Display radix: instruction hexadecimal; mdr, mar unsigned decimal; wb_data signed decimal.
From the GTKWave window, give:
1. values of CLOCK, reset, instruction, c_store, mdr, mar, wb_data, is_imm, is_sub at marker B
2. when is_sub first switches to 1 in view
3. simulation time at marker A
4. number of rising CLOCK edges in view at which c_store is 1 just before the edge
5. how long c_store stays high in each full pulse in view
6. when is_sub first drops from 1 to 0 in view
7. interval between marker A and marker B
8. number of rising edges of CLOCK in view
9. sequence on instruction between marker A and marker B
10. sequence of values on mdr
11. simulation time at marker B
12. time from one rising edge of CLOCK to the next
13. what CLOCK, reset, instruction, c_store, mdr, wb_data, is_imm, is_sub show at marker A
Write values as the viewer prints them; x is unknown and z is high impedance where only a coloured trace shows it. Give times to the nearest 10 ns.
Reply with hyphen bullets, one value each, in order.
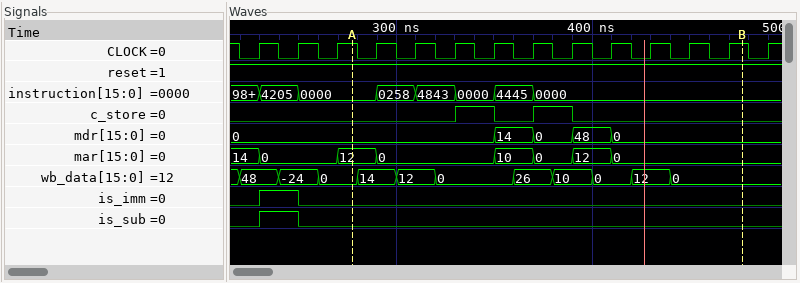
- CLOCK=1, reset=1, instruction=0000, c_store=0, mdr=0, mar=0, wb_data=0, is_imm=0, is_sub=0
- 230 ns
- 280 ns
- 2
- 20 ns, 20 ns
- 250 ns
- 200 ns
- 14
- 0000, 0258, 4843, 0000, 4445, 0000
- 0, 14, 0, 48, 0
- 480 ns
- 20 ns
- CLOCK=1, reset=1, instruction=0000, c_store=0, mdr=0, wb_data=0, is_imm=0, is_sub=0
